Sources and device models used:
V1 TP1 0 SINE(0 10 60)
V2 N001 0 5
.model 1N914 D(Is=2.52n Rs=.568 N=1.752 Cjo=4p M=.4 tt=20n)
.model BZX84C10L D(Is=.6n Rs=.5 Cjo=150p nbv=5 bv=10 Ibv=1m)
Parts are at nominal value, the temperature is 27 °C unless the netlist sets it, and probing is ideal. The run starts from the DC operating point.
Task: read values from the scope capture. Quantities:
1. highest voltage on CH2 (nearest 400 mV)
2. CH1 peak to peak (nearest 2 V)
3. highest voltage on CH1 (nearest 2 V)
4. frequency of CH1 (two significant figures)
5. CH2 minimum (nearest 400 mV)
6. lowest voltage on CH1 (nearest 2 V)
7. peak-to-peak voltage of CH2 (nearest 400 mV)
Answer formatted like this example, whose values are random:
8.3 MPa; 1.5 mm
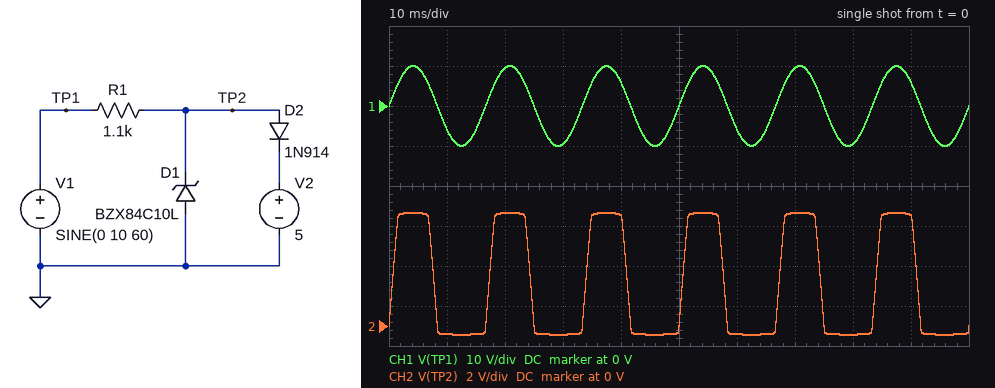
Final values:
5.6 V; 20 V; 10 V; 60 Hz; -400 mV; -10 V; 6.0 V
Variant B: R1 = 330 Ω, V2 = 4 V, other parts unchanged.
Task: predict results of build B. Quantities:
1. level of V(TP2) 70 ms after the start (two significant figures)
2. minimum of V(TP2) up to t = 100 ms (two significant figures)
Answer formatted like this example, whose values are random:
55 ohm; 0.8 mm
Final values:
4.7 V; -470 mV
